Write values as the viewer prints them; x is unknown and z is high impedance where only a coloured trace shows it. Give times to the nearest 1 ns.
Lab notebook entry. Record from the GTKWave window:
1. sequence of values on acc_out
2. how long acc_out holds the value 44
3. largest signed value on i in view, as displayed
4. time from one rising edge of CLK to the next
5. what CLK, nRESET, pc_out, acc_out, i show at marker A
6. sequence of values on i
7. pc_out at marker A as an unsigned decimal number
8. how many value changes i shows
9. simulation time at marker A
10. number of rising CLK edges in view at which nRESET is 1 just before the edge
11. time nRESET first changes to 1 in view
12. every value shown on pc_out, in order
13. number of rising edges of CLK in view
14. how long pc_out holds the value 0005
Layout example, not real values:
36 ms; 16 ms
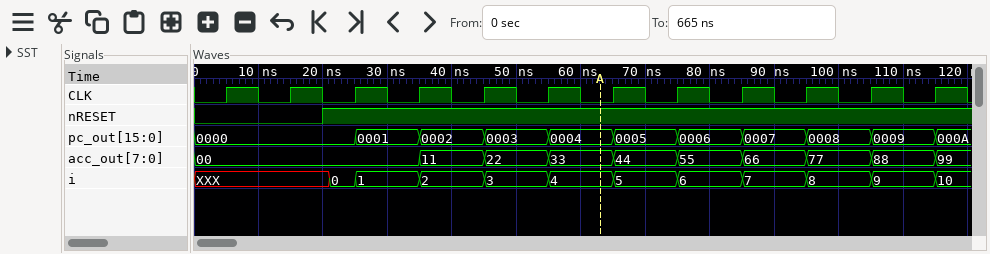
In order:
00, 11, 22, 33, 44, 55, 66, 77, 88, 99; 10 ns; 10; 10 ns; CLK=0, nRESET=1, pc_out=0004, acc_out=33, i=4; XXX, 0, 1, 2, 3, 4, 5, 6, 7, 8, 9, 10; 4; 11; 63 ns; 10; 20 ns; 0000, 0001, 0002, 0003, 0004, 0005, 0006, 0007, 0008, 0009, 000A; 12; 10 ns
